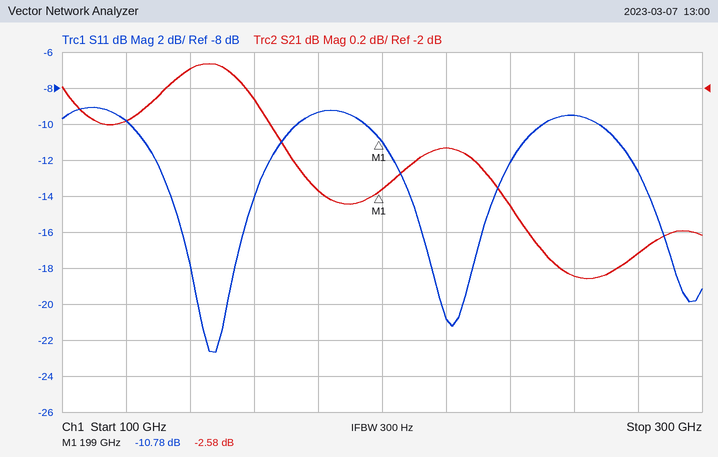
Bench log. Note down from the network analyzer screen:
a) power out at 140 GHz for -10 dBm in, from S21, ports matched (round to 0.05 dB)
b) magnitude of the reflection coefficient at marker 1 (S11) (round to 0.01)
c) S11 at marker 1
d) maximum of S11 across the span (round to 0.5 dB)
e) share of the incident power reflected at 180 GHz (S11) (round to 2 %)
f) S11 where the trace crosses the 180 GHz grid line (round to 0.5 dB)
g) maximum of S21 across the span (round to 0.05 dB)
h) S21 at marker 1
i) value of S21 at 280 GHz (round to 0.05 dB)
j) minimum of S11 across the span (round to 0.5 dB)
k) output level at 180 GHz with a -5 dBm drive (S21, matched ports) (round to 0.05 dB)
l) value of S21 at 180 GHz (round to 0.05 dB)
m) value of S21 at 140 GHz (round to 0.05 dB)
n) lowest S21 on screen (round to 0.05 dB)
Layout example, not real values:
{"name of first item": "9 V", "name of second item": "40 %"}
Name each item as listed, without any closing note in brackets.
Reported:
{"power out at 140 GHz for -10 dBm in, from S21, ports matched": "-11.90 dBm", "magnitude of the reflection coefficient at marker 1 (S11)": "0.29", "S11 at marker 1": "-10.78 dB", "maximum of S11 across the span": "-9.0 dB", "share of the incident power reflected at 180 GHz (S11)": "12 %", "S11 where the trace crosses the 180 GHz grid line": "-9.5 dB", "maximum of S21 across the span": "-1.85 dB", "S21 at marker 1": "-2.58 dB", "value of S21 at 280 GHz": "-2.90 dB", "minimum of S11 across the span": "-22.5 dB", "output level at 180 GHz with a -5 dBm drive (S21, matched ports)": "-7.55 dBm", "value of S21 at 180 GHz": "-2.55 dB", "value of S21 at 140 GHz": "-1.90 dB", "lowest S21 on screen": "-3.05 dB"}
